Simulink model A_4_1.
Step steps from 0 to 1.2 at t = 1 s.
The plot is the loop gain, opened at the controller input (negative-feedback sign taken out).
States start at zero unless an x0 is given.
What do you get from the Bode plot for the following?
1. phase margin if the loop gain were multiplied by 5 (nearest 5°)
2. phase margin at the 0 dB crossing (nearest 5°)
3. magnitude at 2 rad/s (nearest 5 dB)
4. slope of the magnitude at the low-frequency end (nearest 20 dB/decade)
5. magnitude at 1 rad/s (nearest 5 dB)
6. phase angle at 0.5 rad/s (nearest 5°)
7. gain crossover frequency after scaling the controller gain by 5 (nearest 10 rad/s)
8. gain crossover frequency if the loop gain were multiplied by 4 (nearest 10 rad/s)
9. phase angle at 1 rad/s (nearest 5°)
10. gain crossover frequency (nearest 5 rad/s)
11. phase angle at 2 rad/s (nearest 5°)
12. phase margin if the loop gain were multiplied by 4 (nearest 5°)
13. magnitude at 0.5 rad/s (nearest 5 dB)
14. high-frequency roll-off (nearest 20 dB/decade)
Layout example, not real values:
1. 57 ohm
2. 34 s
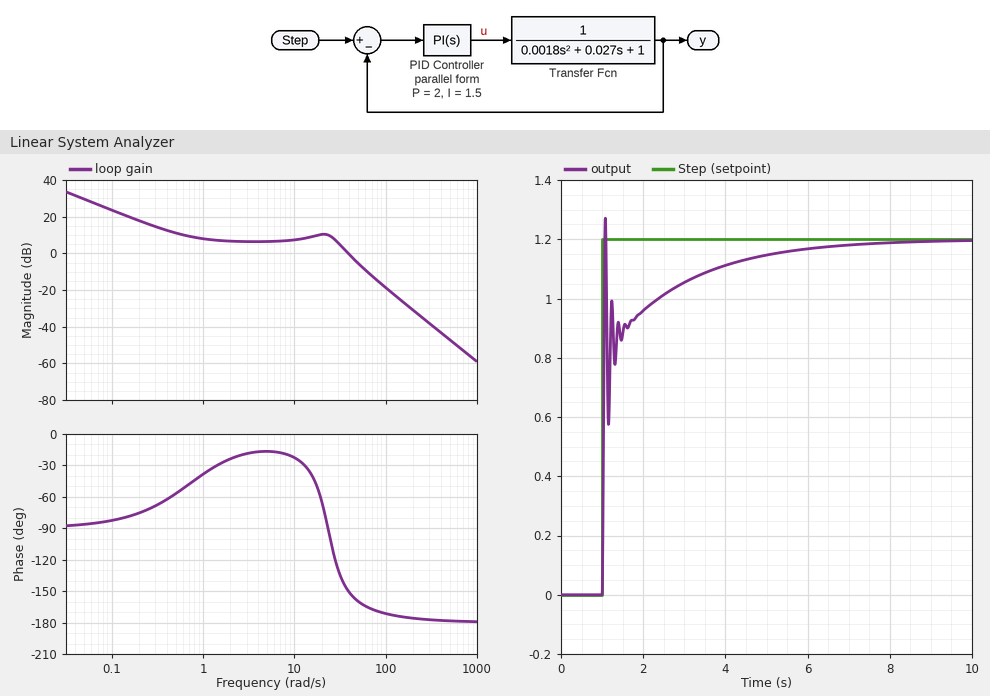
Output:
1. 10°
2. 30°
3. 5 dB
4. -20 dB/decade
5. 10 dB
6. -55°
7. 80 rad/s
8. 70 rad/s
9. -40°
10. 40 rad/s
11. -25°
12. 15°
13. 10 dB
14. -40 dB/decade
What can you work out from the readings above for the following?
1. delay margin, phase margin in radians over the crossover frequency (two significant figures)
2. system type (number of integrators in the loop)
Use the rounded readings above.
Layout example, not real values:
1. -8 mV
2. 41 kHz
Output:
1. 0.013 s
2. 1
